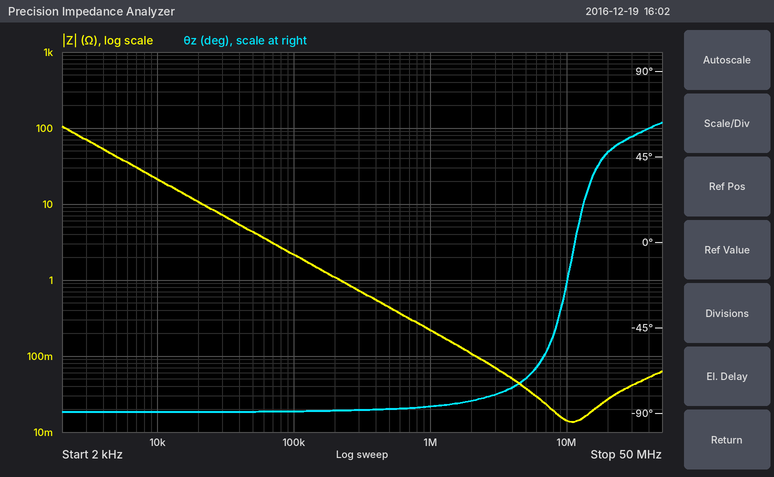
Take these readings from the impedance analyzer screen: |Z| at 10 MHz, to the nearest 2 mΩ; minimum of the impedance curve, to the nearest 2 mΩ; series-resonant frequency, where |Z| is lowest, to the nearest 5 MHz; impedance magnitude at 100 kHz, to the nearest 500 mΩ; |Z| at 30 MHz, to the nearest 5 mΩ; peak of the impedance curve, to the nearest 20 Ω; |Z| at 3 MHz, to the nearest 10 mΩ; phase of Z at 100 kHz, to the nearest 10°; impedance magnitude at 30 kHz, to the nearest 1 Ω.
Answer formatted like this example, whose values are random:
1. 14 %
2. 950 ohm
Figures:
1. 14 mΩ
2. 14 mΩ
3. 10 MHz
4. 2.0 Ω
5. 40 mΩ
6. 100 Ω
7. 70 mΩ
8. -90°
9. 7 Ω
